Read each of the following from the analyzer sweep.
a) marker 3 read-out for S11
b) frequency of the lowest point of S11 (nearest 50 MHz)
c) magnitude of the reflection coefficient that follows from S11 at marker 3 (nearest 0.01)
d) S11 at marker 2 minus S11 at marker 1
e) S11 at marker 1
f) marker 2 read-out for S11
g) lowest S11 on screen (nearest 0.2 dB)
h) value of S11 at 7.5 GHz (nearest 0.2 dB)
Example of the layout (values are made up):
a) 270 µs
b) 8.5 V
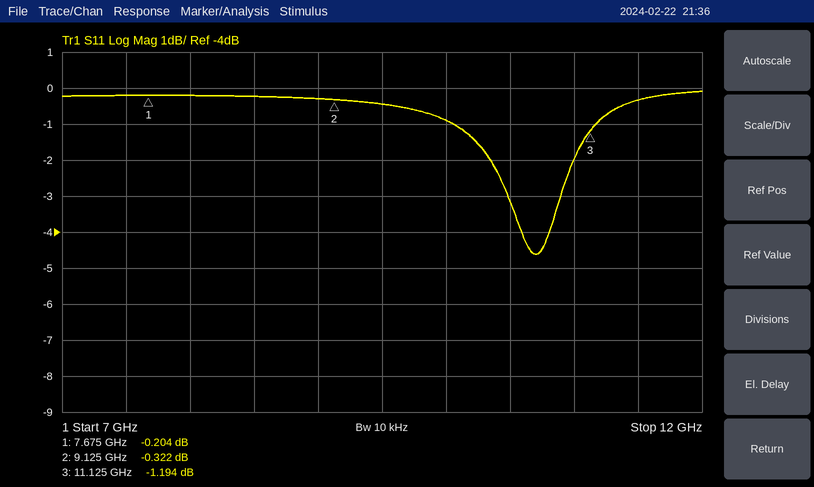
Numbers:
a) -1.194 dB
b) 10.70 GHz
c) 0.87
d) -0.118 dB
e) -0.204 dB
f) -0.322 dB
g) -4.6 dB
h) -0.2 dB
